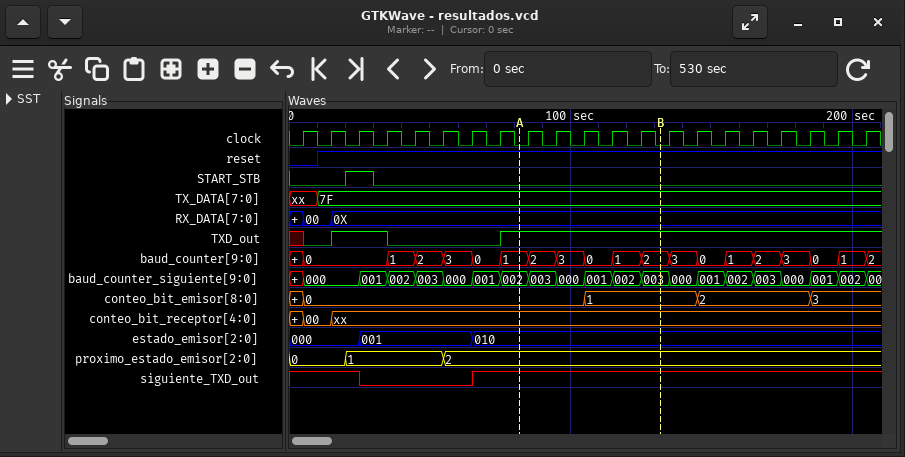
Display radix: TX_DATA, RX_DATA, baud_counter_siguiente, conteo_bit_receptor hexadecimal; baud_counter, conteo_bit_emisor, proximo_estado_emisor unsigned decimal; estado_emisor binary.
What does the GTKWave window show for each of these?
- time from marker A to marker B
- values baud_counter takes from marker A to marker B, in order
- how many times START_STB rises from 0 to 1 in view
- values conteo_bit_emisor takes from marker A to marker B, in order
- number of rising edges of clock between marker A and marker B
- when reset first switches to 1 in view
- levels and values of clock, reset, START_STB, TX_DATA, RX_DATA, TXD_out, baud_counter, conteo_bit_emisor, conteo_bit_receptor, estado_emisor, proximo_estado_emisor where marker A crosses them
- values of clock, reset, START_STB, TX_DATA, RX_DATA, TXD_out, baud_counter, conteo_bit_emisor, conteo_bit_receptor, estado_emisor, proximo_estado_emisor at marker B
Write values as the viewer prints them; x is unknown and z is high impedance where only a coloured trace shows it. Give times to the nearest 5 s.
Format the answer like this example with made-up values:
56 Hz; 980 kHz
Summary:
50 s; 1, 2, 3, 0, 1, 2; 1; 0, 1; 5; 10 s; clock=0, reset=1, START_STB=0, TX_DATA=7F, RX_DATA=0X, TXD_out=1, baud_counter=1, conteo_bit_emisor=0, conteo_bit_receptor=xx, estado_emisor=010, proximo_estado_emisor=2; clock=0, reset=1, START_STB=0, TX_DATA=7F, RX_DATA=0X, TXD_out=1, baud_counter=2, conteo_bit_emisor=1, conteo_bit_receptor=xx, estado_emisor=010, proximo_estado_emisor=2
